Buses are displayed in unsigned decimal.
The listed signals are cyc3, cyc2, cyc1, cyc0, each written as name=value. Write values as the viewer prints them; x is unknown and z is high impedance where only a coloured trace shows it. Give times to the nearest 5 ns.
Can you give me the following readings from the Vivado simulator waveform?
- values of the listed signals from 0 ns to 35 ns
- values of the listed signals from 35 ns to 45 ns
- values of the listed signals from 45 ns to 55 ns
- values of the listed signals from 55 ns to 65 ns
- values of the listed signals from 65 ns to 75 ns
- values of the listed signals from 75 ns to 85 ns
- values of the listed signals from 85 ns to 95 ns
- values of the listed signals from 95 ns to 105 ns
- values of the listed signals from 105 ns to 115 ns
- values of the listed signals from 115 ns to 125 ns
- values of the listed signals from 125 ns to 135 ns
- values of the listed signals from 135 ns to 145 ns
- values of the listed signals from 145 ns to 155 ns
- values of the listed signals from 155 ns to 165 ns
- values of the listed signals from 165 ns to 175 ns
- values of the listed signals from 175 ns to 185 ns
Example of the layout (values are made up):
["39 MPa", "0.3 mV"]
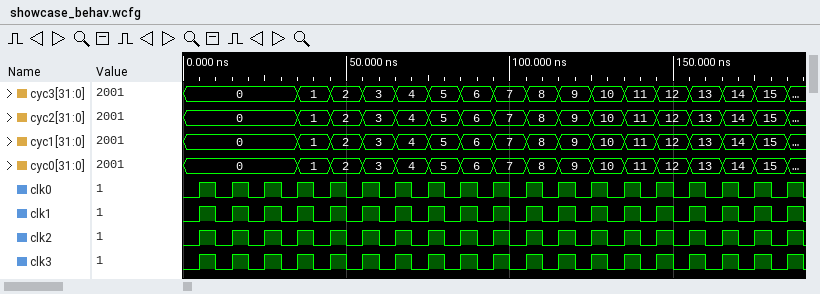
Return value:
["cyc3=0, cyc2=0, cyc1=0, cyc0=0", "cyc3=1, cyc2=1, cyc1=1, cyc0=1", "cyc3=2, cyc2=2, cyc1=2, cyc0=2", "cyc3=3, cyc2=3, cyc1=3, cyc0=3", "cyc3=4, cyc2=4, cyc1=4, cyc0=4", "cyc3=5, cyc2=5, cyc1=5, cyc0=5", "cyc3=6, cyc2=6, cyc1=6, cyc0=6", "cyc3=7, cyc2=7, cyc1=7, cyc0=7", "cyc3=8, cyc2=8, cyc1=8, cyc0=8", "cyc3=9, cyc2=9, cyc1=9, cyc0=9", "cyc3=10, cyc2=10, cyc1=10, cyc0=10", "cyc3=11, cyc2=11, cyc1=11, cyc0=11", "cyc3=12, cyc2=12, cyc1=12, cyc0=12", "cyc3=13, cyc2=13, cyc1=13, cyc0=13", "cyc3=14, cyc2=14, cyc1=14, cyc0=14", "cyc3=15, cyc2=15, cyc1=15, cyc0=15"]
